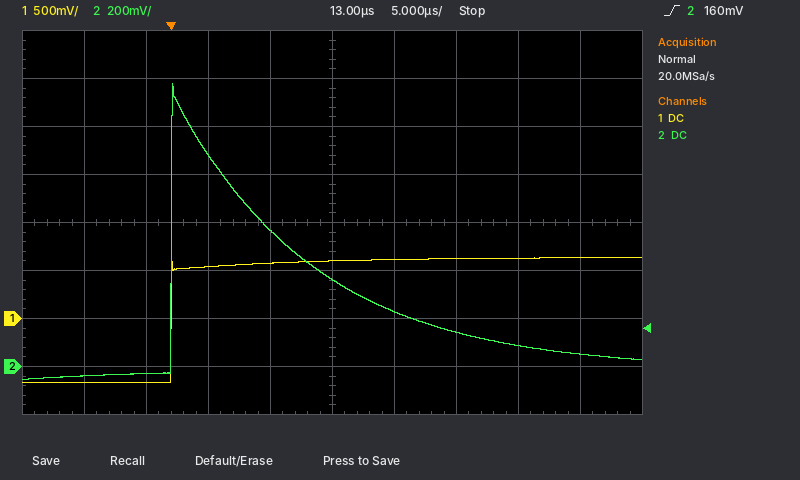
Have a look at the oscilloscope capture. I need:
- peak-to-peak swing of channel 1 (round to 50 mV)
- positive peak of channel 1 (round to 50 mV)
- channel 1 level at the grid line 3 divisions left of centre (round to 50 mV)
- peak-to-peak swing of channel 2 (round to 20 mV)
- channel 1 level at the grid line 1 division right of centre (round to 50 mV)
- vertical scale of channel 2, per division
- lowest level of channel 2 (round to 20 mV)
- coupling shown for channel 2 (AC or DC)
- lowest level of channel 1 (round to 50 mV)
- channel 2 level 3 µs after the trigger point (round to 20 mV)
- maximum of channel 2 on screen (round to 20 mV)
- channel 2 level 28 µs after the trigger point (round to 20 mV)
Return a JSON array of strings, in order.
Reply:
["1.30 V", "650 mV", "-650 mV", "1.24 V", "600 mV", "200 mV", "-60 mV", "DC", "-650 mV", "880 mV", "1.18 V", "80 mV"]
